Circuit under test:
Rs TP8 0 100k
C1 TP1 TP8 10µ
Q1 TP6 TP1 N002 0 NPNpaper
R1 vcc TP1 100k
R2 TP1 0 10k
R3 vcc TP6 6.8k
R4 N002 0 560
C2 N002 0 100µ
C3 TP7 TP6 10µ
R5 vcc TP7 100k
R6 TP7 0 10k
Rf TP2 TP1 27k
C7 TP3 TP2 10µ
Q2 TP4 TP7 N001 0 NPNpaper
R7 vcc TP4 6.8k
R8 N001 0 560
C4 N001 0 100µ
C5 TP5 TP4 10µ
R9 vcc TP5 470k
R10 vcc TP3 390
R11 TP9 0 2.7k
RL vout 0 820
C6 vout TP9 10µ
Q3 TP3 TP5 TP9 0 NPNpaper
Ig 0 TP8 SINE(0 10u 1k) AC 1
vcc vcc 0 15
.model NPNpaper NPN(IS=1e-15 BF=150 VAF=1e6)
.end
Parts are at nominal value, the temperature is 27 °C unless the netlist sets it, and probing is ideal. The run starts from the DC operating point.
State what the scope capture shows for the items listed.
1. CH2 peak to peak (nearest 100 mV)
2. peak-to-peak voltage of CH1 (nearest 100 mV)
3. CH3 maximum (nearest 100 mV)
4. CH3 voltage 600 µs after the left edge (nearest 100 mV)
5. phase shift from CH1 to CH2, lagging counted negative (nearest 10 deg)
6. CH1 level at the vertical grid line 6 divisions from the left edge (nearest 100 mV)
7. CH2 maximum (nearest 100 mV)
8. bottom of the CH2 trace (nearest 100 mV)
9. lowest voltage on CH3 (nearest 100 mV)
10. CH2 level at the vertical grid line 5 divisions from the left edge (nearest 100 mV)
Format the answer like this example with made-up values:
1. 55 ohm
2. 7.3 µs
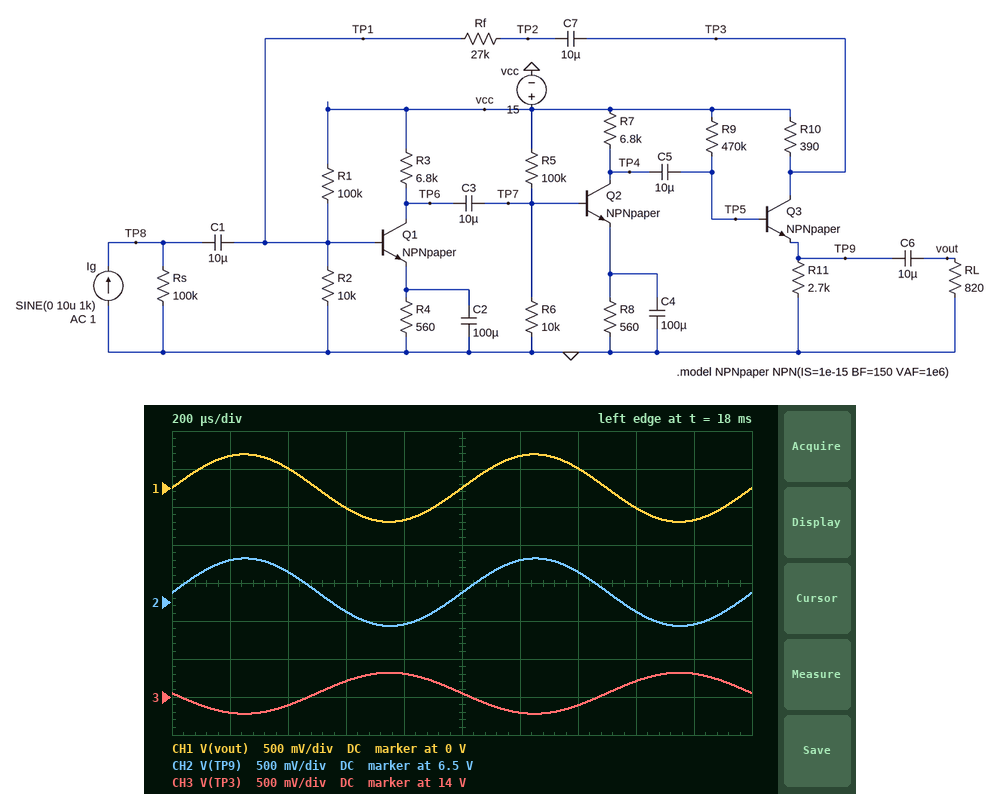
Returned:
1. 900 mV
2. 900 mV
3. 14.3 V
4. 14.2 V
5. 0 deg
6. 400 mV
7. 7.1 V
8. 6.2 V
9. 13.8 V
10. 6.6 V
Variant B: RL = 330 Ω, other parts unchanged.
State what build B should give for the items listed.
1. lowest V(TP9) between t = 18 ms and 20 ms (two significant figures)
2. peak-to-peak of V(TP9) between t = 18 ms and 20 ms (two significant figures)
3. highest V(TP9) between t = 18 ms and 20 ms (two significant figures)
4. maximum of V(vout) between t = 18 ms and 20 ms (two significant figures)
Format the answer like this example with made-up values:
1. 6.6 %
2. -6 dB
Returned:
1. 6.4 V
2. 420 mV
3. 6.8 V
4. 210 mV
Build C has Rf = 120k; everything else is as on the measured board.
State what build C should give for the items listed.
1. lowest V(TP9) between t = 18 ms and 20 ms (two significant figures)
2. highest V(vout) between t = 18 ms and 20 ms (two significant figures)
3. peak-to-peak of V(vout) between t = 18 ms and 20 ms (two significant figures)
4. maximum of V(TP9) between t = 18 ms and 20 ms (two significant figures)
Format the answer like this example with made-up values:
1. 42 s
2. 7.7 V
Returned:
1. 5.2 V
2. 2.0 V
3. 3.6 V
4. 8.9 V
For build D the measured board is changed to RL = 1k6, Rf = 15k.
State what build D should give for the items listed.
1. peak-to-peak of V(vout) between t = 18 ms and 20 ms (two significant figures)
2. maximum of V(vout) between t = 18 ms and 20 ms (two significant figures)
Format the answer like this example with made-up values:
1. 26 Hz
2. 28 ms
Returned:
1. 800 mV
2. 400 mV
